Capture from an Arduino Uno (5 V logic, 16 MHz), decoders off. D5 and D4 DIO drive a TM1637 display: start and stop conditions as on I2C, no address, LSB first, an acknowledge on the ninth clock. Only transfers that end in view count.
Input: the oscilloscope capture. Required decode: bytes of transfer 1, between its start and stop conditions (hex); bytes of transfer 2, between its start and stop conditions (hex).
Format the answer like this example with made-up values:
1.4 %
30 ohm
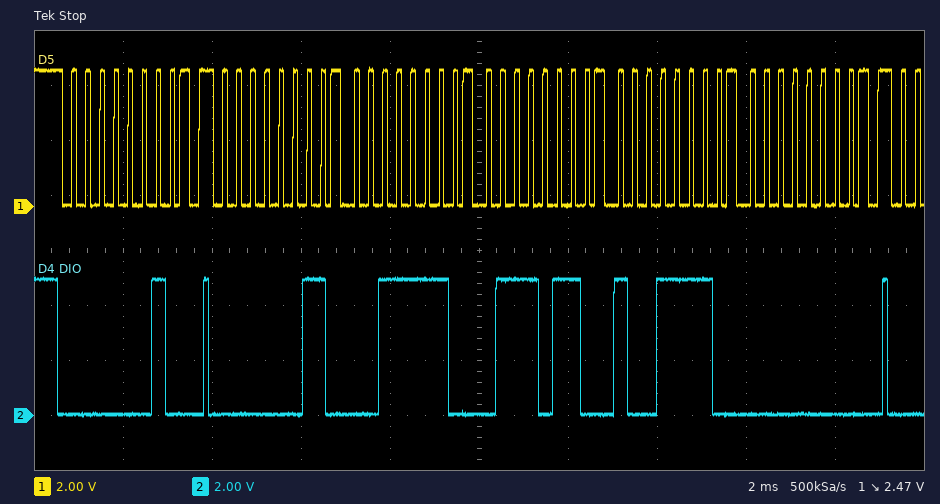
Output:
40
C0 7C 6E 79 00
